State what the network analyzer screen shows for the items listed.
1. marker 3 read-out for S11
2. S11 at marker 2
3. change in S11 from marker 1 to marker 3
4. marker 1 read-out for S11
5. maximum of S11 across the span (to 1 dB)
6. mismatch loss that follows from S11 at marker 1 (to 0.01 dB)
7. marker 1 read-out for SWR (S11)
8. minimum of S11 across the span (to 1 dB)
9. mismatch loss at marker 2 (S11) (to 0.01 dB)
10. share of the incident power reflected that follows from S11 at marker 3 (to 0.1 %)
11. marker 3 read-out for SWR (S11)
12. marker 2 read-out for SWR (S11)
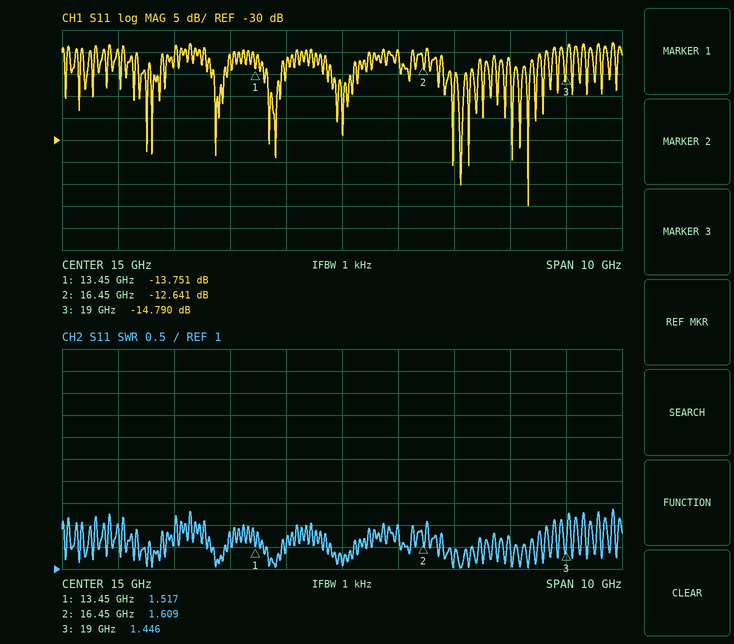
-14.790 dB
-12.641 dB
-1.039 dB
-13.751 dB
-8 dB
0.19 dB
1.517
-45 dB
0.24 dB
3.3 %
1.446
1.609
